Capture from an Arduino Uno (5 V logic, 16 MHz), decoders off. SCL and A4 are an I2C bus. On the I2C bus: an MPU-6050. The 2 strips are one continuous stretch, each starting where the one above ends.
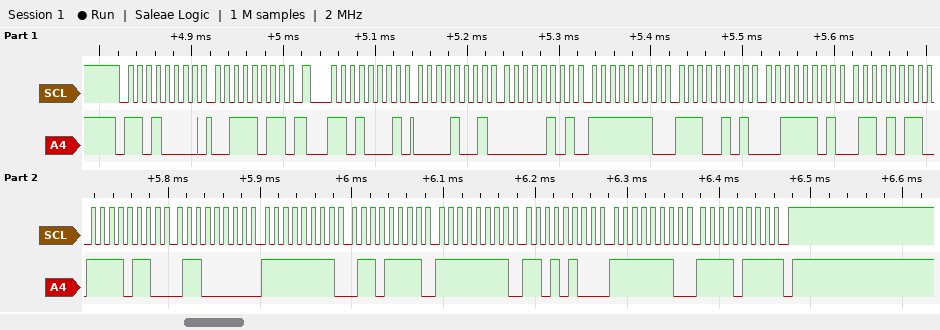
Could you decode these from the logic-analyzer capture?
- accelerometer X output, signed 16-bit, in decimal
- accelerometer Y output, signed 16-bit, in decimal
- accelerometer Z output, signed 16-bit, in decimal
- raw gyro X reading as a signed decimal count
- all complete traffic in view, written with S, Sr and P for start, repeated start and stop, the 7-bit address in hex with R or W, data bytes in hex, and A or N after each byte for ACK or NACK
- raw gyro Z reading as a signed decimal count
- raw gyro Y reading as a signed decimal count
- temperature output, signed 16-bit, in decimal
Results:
2309
-283
15723
-145
S 68W A 3B A Sr 68R A 09 A 05 A FE A E5 A 3D A 6B A F6 A 60 A FF A 6F A FF A D4 A FE A F7 N P
-265
-44
-2464
